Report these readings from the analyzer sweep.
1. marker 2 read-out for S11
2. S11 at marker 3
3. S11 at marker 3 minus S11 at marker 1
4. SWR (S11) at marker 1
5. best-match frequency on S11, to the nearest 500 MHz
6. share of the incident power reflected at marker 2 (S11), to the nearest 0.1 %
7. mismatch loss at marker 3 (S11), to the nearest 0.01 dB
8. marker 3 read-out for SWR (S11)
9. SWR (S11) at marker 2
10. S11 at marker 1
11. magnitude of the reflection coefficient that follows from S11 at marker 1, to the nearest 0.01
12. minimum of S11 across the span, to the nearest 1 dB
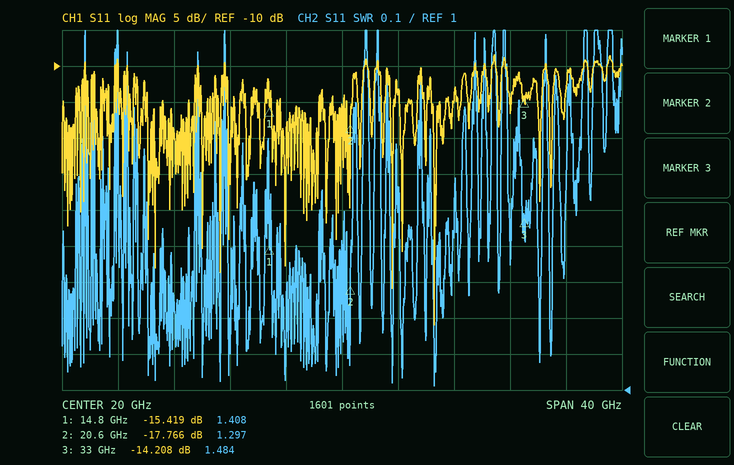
-17.766 dB
-14.208 dB
1.211 dB
1.408
26.5 GHz
1.7 %
0.17 dB
1.484
1.297
-15.419 dB
0.17
-46 dB
